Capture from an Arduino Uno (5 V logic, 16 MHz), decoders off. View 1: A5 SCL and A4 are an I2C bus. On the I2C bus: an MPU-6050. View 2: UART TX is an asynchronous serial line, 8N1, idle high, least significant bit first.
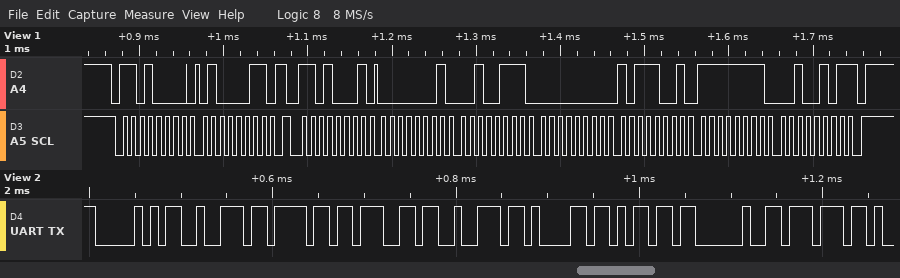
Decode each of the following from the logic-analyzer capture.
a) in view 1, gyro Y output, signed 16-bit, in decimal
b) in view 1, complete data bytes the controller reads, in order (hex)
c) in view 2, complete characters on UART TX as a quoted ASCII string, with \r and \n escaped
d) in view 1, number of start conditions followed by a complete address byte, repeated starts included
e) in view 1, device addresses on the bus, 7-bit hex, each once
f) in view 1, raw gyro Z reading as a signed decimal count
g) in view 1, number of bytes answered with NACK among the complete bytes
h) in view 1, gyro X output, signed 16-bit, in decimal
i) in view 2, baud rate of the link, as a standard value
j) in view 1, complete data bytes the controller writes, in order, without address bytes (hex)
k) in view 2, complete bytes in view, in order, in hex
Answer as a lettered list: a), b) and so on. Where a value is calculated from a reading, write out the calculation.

a) 0x00B9 = 185
b) 01 27 00 B9 FF 25
c) "Program w"
d) 2
e) 0x68
f) 0xFF25 = -219
g) 1
h) 0x0127 = 295
i) 115200 baud
j) 43
k) 50 72 6F 67 72 61 6D 20 77
